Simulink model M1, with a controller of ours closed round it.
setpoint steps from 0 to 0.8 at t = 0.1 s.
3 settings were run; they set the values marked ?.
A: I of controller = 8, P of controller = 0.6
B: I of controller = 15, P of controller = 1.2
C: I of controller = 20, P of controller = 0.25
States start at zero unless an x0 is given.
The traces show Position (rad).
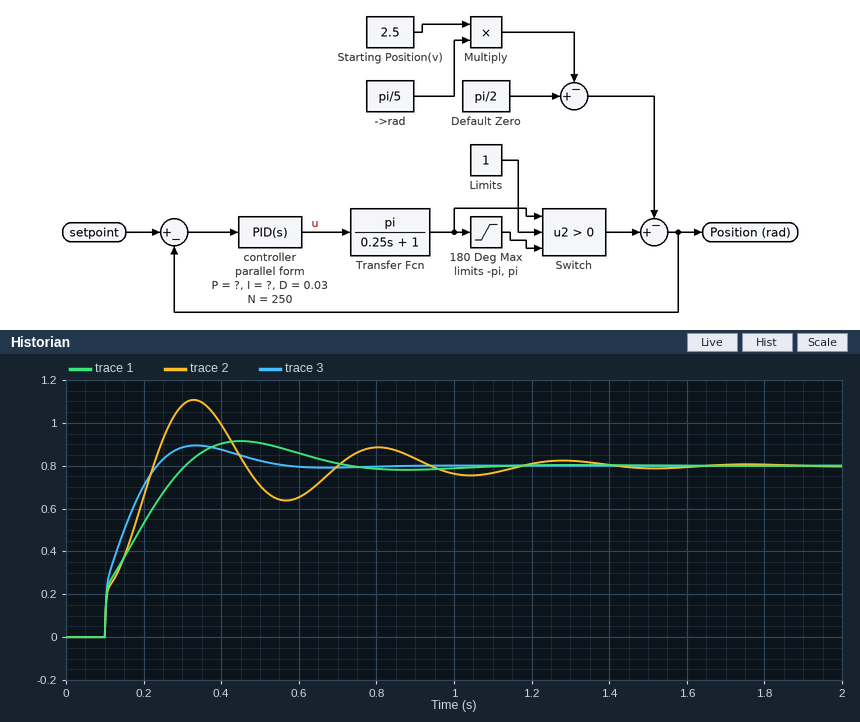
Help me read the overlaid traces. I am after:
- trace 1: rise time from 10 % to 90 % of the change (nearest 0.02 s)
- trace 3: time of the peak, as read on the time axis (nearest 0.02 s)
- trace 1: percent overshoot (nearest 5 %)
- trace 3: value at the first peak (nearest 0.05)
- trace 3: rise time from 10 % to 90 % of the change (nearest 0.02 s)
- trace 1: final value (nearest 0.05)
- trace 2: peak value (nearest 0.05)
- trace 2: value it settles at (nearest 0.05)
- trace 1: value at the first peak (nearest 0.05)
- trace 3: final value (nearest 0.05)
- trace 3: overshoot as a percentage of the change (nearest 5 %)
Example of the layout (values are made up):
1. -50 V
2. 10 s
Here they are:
1. 0.16 s
2. 0.34 s
3. 15 %
4. 0.90
5. 0.10 s
6. 0.80
7. 1.10
8. 0.80
9. 0.90
10. 0.80
11. 10 %
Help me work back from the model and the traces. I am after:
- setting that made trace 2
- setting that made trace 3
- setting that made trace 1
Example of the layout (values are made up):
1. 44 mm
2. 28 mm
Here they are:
1. C
2. B
3. A
